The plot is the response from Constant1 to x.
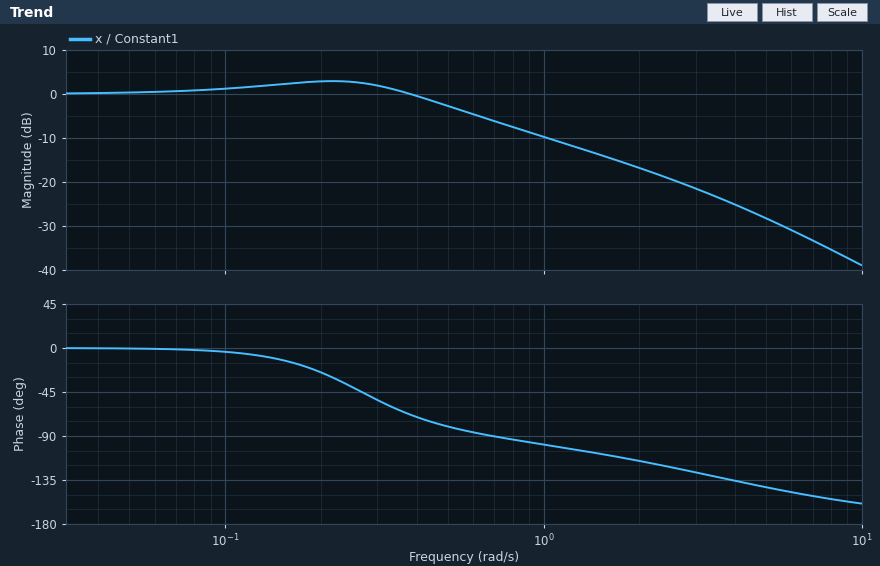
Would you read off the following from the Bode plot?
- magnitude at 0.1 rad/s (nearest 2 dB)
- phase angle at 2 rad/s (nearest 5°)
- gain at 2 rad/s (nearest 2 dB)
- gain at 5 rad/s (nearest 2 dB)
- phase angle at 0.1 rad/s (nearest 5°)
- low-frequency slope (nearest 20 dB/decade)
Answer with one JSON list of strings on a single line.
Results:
["2 dB", "-115°", "-16 dB", "-28 dB", "-5°", "0 dB/decade"]
